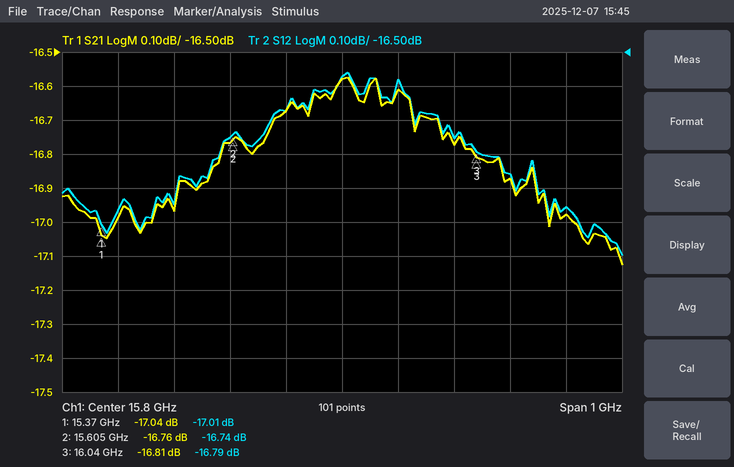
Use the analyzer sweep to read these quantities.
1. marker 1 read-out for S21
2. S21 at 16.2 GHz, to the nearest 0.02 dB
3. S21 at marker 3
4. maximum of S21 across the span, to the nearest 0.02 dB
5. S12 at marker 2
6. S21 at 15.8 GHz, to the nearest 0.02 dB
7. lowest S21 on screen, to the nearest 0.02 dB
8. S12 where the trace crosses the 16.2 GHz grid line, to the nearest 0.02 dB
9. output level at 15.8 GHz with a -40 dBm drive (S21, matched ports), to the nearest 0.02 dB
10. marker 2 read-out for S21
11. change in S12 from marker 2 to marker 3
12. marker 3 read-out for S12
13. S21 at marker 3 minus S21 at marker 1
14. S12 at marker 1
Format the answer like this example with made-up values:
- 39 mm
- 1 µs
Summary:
- -17.04 dB
- -16.98 dB
- -16.81 dB
- -16.58 dB
- -16.74 dB
- -16.58 dB
- -17.12 dB
- -16.96 dB
- -56.58 dBm
- -16.76 dB
- -0.05 dB
- -16.79 dB
- 0.23 dB
- -17.01 dB
